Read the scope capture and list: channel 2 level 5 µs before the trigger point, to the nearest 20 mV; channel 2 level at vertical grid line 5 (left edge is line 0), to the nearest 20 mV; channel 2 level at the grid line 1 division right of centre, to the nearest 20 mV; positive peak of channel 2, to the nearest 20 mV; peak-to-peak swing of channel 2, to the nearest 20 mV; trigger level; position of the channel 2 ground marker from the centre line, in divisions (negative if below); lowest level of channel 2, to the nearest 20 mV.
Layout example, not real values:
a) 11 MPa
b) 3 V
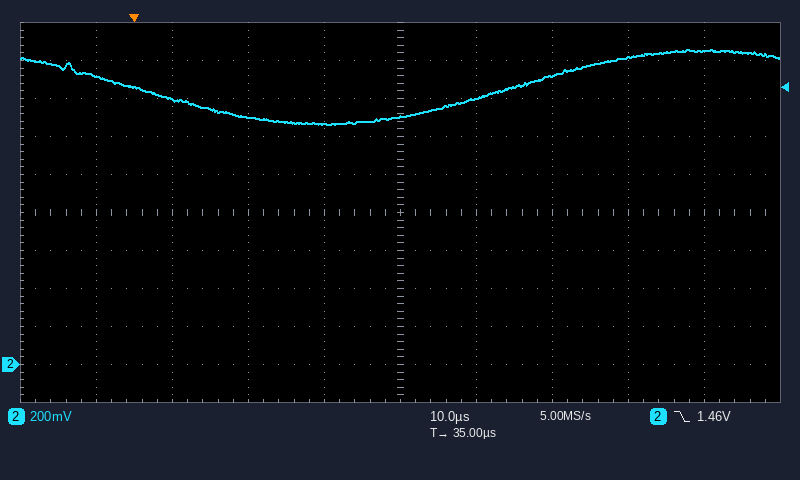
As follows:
a) 1.52 V
b) 1.30 V
c) 1.40 V
d) 1.66 V
e) 400 mV
f) 1.46 V
g) -4.0 div
h) 1.26 V
